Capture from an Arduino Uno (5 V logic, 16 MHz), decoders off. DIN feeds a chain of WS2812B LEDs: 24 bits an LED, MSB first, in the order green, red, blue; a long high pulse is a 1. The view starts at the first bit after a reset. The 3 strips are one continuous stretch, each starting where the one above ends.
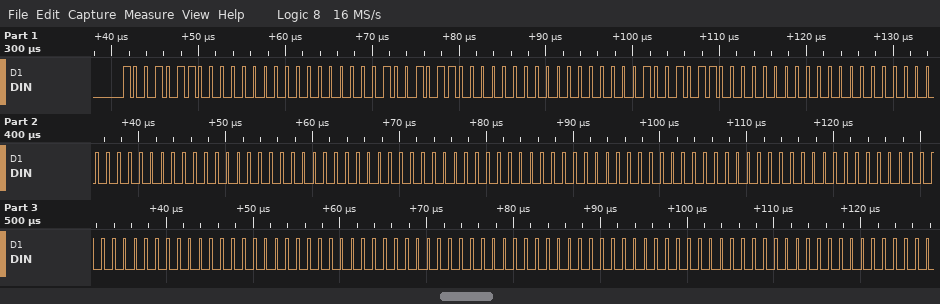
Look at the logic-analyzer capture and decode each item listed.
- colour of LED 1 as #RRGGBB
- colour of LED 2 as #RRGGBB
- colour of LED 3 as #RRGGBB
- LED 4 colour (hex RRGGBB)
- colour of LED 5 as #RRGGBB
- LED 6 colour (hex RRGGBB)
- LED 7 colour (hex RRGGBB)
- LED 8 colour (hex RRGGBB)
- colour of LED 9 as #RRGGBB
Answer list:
#009600
#009600
#009600
#000000
#000000
#000000
#000000
#000000
#000000
